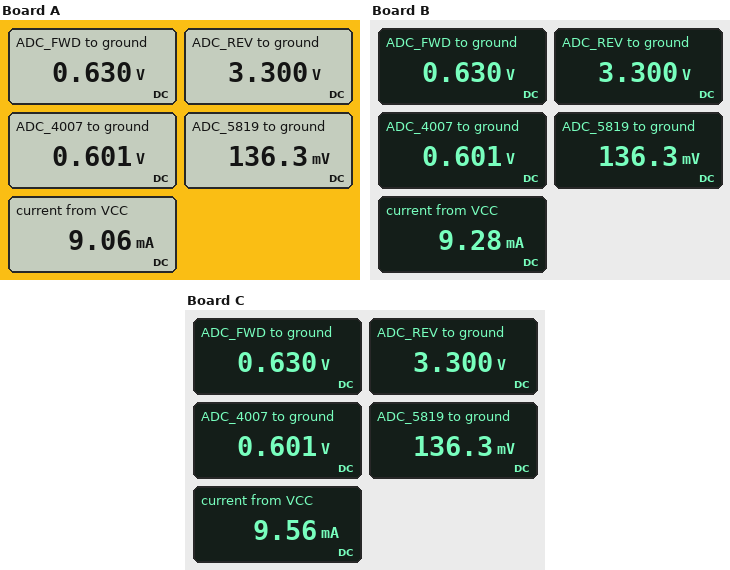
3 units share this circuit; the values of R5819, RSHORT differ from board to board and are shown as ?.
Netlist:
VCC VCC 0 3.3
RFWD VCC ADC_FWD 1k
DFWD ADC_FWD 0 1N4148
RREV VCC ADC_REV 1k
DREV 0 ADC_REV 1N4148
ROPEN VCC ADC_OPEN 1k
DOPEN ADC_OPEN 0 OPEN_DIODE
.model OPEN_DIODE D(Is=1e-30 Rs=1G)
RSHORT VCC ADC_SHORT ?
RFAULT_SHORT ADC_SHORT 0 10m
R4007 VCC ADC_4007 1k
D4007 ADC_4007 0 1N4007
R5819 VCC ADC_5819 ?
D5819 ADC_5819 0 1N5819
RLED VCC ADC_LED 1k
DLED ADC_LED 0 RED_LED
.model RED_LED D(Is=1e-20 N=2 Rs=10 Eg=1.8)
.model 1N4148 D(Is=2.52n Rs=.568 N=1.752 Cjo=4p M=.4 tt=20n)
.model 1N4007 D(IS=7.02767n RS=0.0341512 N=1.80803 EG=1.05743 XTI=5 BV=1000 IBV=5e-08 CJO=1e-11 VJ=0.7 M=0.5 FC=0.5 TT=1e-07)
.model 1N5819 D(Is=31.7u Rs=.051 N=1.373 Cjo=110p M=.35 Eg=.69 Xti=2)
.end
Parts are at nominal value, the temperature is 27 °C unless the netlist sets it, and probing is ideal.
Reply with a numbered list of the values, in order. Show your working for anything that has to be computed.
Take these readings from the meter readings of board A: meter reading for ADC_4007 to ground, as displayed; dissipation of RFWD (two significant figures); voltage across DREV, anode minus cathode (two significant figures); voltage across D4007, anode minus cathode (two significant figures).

1. 0.601 V
2. (3.3 V - 630 mV)^2 / 1 kΩ = 7.1 mW
3. 0 V - 3.3 V = -3.3 V
4. 601 mV = 600 mV
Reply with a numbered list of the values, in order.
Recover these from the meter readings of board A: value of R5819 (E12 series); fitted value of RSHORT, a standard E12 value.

1. 2.2 kΩ
2. 3.3 kΩ
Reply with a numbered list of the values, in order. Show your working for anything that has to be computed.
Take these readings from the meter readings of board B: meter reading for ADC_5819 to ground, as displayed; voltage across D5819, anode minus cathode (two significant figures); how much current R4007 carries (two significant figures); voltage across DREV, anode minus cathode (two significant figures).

1. 136.3 mV
2. 136.3 mV = 140 mV
3. (3.3 V - 601 mV) / 1 kΩ = 2.7 mA
4. 0 V - 3.3 V = -3.3 V
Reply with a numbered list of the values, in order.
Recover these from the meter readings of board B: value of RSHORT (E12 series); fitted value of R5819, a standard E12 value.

1. 2.7 kΩ
2. 2.2 kΩ
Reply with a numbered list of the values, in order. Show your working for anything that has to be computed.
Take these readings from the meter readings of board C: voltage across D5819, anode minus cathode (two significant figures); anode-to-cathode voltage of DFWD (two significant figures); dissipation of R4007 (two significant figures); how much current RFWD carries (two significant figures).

1. 136.3 mV = 140 mV
2. 630 mV = 630 mV
3. (3.3 V - 601 mV)^2 / 1 kΩ = 7.3 mW
4. (3.3 V - 630 mV) / 1 kΩ = 2.7 mA
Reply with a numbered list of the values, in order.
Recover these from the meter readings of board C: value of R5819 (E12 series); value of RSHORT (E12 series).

1. 2.2 kΩ
2. 2.2 kΩ
